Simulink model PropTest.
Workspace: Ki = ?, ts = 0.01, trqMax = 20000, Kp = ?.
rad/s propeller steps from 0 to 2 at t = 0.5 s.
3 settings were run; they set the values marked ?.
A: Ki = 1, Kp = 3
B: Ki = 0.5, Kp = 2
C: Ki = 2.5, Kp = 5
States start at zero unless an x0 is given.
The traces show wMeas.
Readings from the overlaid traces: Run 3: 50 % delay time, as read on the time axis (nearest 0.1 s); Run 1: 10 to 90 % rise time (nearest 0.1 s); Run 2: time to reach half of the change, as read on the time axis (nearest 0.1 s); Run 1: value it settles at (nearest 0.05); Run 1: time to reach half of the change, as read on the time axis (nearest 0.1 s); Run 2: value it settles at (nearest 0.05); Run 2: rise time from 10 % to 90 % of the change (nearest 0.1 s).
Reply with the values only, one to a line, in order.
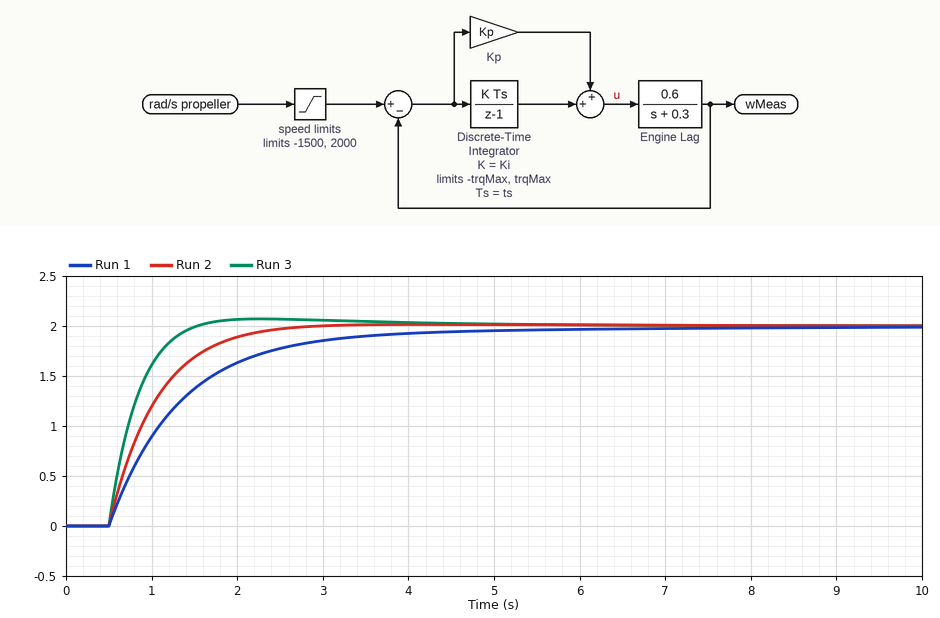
0.7 s
2.0 s
0.9 s
2.00
1.1 s
2.00
1.2 s
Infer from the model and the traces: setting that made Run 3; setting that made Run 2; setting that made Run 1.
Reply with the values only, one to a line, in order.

C
A
B
